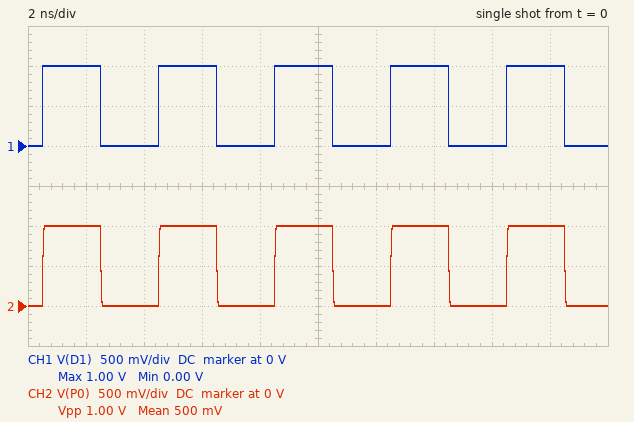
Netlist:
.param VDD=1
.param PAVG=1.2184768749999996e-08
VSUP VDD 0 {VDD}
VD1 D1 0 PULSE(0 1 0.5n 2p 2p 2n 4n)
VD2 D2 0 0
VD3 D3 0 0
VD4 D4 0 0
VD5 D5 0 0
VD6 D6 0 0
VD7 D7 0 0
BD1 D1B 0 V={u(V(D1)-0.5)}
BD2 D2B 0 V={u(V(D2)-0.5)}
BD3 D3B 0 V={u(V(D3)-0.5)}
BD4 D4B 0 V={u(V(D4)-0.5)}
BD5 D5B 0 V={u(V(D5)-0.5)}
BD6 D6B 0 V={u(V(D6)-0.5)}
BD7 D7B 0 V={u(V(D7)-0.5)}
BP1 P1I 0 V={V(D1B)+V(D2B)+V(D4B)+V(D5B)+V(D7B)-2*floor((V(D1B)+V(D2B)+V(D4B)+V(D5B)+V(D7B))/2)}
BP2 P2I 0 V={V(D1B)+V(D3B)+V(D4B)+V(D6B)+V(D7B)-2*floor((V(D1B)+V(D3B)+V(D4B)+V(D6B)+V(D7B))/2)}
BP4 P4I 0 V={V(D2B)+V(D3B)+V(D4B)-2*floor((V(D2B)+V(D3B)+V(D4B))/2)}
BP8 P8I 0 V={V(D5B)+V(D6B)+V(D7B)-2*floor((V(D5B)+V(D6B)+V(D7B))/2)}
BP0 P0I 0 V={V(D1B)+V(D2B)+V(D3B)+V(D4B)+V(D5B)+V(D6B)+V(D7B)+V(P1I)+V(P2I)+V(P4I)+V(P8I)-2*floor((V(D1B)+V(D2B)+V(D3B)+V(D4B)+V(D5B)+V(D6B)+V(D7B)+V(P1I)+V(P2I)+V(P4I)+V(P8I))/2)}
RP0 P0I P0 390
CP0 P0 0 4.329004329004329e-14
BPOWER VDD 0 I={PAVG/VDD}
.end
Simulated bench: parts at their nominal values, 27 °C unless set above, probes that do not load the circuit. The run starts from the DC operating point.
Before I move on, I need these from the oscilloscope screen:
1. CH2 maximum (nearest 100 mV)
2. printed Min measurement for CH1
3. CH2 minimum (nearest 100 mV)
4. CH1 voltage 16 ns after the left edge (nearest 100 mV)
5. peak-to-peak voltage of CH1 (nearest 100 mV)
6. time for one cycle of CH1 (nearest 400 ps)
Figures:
1.0 V
0.00 V
0 V
0 V
1.0 V
4.0 ns
